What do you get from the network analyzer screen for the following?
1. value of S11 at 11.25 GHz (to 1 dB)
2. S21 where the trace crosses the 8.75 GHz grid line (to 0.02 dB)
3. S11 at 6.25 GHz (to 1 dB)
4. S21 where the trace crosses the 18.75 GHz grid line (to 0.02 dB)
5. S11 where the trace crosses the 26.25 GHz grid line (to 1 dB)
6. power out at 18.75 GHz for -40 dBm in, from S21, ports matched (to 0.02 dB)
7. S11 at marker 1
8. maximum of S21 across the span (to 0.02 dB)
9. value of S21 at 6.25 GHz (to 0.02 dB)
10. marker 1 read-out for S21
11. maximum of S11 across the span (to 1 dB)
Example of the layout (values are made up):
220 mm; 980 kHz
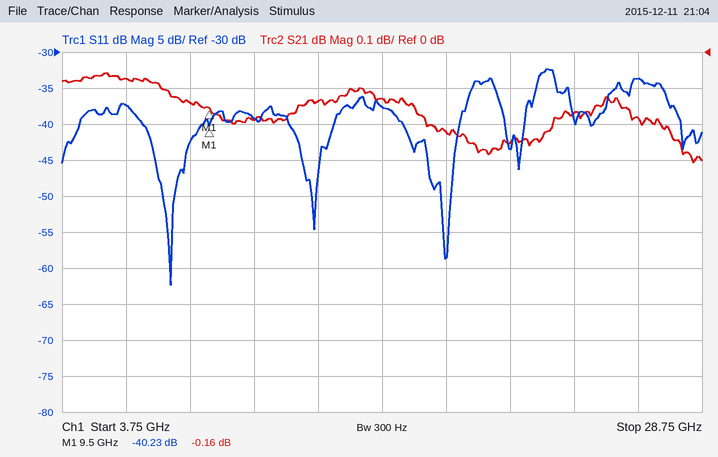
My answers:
-39 dB; -0.14 dB; -37 dB; -0.22 dB; -34 dB; -40.22 dBm; -40.23 dB; -0.06 dB; -0.08 dB; -0.16 dB; -32 dB
